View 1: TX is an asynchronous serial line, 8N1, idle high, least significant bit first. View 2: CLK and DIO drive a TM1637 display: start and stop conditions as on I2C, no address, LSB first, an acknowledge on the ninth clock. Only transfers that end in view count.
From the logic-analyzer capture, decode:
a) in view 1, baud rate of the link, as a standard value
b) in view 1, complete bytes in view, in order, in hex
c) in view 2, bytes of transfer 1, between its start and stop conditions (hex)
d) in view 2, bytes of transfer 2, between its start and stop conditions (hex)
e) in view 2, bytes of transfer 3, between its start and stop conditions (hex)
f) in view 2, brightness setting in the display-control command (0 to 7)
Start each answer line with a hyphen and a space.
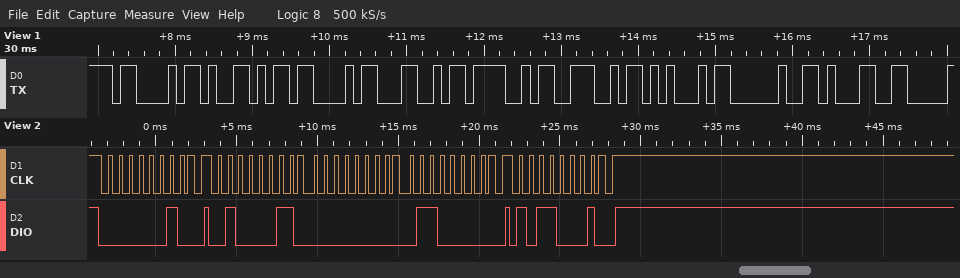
- 9600 baud
- 0x43 0x59 0x43 0x4C 0x4F 0x4E 0x45 0x20 0x31
- 40
- C2 00 06
- 8D
- 5
